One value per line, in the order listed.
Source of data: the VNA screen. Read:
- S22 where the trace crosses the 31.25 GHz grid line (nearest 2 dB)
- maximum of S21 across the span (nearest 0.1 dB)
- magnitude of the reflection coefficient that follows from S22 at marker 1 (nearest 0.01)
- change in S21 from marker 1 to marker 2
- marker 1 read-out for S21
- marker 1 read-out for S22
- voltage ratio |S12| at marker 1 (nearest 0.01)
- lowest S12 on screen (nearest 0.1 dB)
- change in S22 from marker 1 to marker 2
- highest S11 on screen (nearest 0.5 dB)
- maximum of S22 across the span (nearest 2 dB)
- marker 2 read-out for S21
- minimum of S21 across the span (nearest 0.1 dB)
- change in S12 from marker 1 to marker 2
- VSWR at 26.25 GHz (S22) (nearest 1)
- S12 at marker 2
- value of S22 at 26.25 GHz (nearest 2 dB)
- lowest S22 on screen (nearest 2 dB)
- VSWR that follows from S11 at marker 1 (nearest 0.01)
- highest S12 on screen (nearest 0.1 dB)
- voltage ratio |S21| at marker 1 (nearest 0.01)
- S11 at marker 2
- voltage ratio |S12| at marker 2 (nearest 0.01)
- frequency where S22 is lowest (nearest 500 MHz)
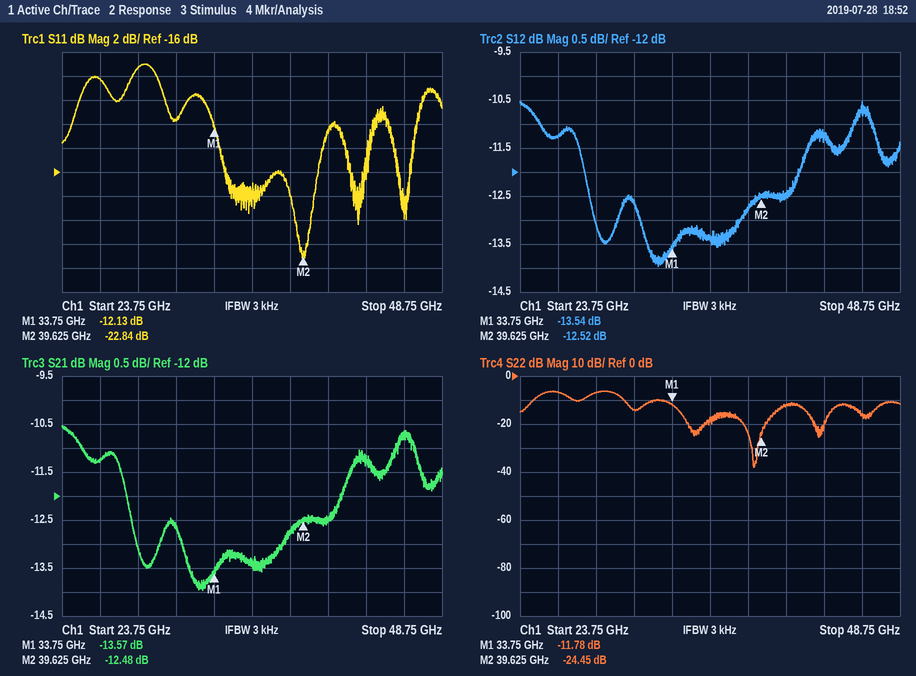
-14 dB
-10.5 dB
0.26
1.09 dB
-13.57 dB
-11.78 dB
0.21
-14.0 dB
-12.67 dB
-7.0 dB
-6 dB
-12.48 dB
-14.0 dB
1.02 dB
3
-12.52 dB
-6 dB
-38 dB
1.66
-10.5 dB
0.21
-22.84 dB
0.24
39.0 GHz
